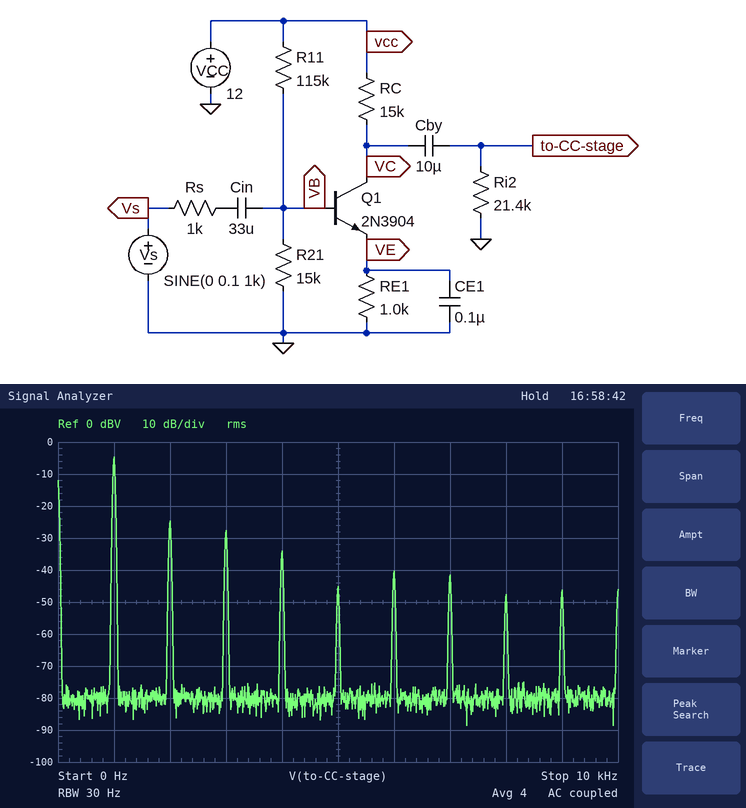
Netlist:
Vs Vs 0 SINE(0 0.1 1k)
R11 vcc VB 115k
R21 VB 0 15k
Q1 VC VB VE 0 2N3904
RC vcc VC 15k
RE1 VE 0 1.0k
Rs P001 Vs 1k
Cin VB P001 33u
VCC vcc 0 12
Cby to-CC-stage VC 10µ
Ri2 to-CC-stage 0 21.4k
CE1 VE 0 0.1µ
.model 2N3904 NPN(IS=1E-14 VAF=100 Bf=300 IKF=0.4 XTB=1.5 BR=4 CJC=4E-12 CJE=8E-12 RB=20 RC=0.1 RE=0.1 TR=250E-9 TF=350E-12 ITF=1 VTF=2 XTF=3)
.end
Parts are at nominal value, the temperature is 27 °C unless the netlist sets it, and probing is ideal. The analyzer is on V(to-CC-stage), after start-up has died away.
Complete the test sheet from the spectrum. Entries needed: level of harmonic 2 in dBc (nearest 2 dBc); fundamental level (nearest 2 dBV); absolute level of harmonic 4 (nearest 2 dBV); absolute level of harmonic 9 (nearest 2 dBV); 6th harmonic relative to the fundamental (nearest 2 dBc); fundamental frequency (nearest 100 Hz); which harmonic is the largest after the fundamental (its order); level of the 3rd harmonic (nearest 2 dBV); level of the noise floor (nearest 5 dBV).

-20 dBc
-4 dBV
-34 dBV
-46 dBV
-36 dBc
1.0 kHz
2
-28 dBV
-80 dBV
